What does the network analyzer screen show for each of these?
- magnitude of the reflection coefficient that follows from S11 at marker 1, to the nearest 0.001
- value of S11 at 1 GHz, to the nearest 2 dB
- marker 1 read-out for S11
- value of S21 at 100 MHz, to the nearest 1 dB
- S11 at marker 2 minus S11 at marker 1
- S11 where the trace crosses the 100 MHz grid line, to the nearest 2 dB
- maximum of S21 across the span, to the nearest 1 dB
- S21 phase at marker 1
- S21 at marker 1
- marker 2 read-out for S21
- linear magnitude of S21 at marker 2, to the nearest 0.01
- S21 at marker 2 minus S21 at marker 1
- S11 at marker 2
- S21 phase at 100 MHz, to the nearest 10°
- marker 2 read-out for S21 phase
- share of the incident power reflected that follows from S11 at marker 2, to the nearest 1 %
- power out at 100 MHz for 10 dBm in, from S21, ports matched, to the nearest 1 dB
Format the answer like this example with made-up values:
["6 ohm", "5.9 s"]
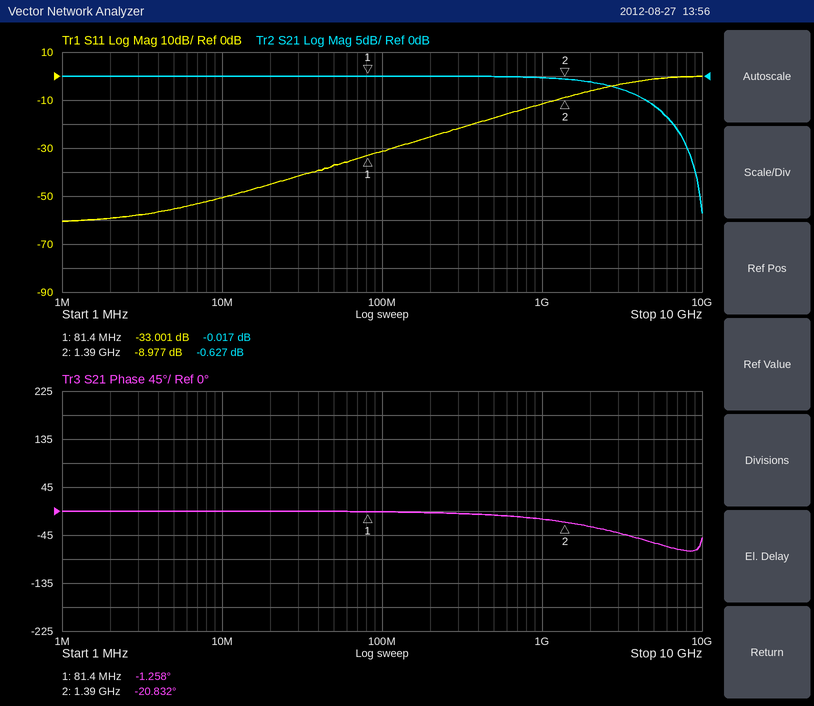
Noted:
["0.022", "-12 dB", "-33.001 dB", "0 dB", "24.024 dB", "-32 dB", "0 dB", "-1.258°", "-0.017 dB", "-0.627 dB", "0.93", "-0.610 dB", "-8.977 dB", "0°", "-20.832°", "13 %", "10 dBm"]
